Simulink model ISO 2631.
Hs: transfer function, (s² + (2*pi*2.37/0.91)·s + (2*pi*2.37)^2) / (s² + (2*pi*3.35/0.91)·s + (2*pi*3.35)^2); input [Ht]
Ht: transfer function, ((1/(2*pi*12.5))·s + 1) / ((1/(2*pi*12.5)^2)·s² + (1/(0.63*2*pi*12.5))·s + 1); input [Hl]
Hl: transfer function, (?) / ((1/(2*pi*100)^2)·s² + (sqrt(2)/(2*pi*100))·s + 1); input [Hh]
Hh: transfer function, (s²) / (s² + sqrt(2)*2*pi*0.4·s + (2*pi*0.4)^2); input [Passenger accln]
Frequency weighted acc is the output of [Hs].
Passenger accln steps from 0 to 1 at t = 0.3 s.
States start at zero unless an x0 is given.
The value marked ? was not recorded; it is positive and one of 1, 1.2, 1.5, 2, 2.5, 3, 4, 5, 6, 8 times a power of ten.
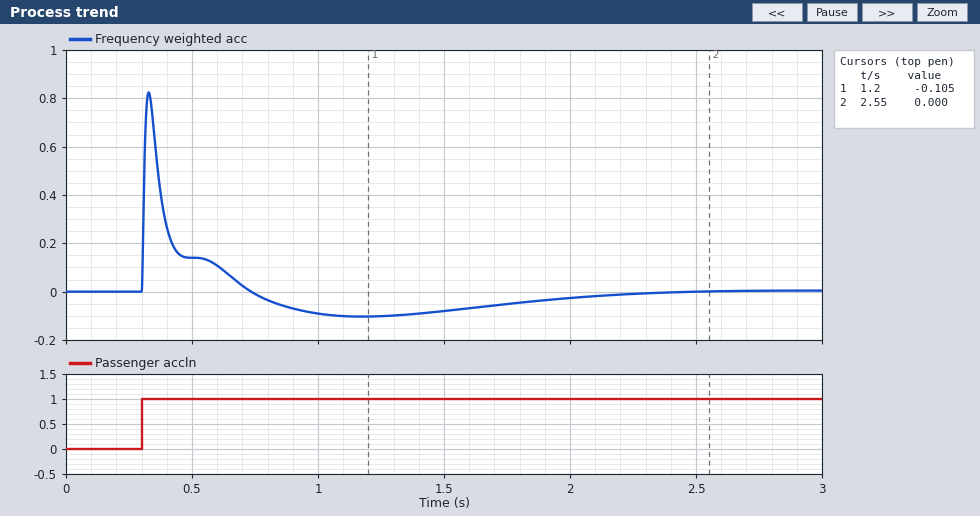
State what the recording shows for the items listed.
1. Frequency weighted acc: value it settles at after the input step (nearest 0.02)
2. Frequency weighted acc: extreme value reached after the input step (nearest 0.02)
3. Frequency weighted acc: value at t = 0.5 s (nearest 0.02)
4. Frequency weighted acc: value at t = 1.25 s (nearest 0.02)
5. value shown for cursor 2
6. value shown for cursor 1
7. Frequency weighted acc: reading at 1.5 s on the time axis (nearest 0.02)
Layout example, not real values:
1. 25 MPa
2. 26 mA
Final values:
1. 0.00
2. 0.82
3. 0.14
4. -0.10
5. 0.000
6. -0.105
7. -0.08
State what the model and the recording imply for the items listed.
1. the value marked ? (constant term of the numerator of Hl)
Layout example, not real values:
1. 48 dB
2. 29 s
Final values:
1. 1
